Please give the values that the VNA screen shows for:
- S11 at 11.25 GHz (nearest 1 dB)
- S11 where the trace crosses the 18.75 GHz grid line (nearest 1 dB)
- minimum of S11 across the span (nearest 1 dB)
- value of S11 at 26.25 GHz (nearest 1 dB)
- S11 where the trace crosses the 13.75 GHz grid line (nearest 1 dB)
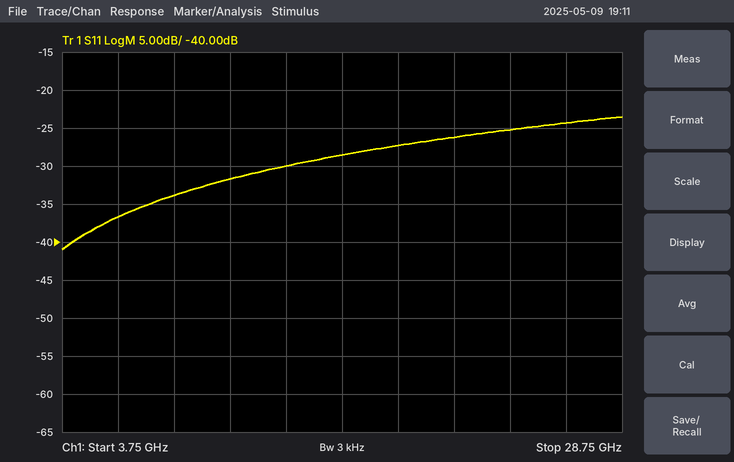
-32 dB
-27 dB
-41 dB
-24 dB
-30 dB
